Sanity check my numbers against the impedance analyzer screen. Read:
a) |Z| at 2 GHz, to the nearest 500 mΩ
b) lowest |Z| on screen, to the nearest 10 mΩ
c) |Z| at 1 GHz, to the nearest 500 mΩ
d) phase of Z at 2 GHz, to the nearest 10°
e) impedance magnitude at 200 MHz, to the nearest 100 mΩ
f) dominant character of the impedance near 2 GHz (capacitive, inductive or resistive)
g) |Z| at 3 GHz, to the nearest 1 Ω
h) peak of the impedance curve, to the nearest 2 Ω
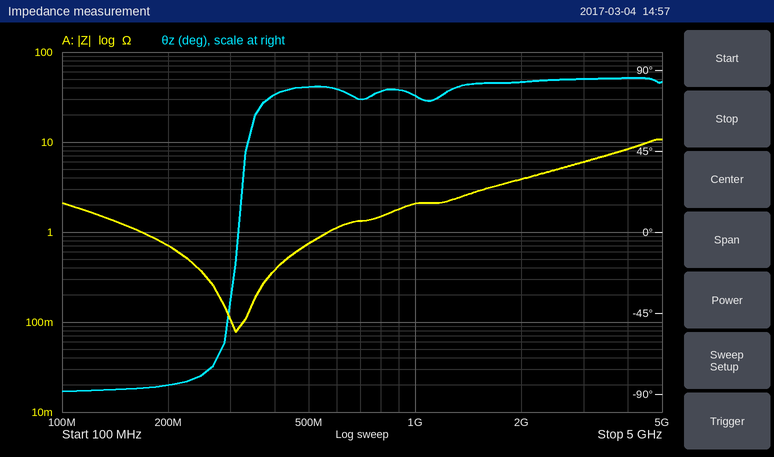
4.0 Ω
80 mΩ
2.0 Ω
80°
700 mΩ
inductive
6 Ω
10 Ω
